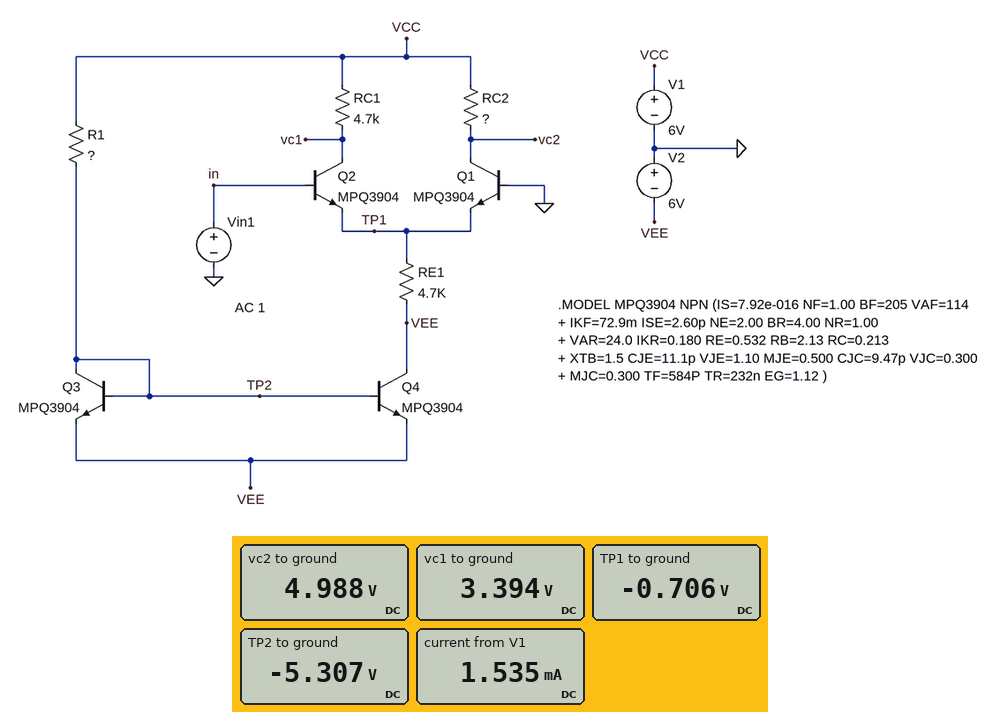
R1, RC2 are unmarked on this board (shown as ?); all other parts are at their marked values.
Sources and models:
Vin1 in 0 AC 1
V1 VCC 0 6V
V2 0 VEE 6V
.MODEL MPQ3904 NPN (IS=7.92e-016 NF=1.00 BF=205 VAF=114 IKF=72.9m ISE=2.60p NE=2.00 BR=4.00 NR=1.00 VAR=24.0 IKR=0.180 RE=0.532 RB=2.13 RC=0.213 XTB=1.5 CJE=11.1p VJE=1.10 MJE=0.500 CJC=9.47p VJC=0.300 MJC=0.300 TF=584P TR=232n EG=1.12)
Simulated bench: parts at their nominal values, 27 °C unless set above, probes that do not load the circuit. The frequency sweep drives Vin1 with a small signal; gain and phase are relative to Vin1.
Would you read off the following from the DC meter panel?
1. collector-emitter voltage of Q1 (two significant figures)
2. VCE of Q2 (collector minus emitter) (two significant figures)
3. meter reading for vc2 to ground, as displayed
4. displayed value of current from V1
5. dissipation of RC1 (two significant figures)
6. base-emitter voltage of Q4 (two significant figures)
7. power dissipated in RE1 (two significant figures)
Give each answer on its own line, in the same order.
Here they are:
5.7 V
4.1 V
4.988 V
1.535 mA
1.4 mW
690 mV
6.0 mW
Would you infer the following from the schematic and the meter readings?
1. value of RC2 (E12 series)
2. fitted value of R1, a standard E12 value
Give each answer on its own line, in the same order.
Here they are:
1.8 kΩ
27 kΩ
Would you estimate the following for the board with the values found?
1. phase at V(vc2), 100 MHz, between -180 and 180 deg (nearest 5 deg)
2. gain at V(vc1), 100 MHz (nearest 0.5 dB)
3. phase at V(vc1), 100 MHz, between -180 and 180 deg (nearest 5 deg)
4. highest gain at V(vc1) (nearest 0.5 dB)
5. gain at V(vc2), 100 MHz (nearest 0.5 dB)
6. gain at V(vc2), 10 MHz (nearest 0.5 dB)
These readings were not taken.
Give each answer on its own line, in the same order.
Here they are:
-80 deg
11.5 dB
75 deg
34.0 dB
12.0 dB
24.5 dB
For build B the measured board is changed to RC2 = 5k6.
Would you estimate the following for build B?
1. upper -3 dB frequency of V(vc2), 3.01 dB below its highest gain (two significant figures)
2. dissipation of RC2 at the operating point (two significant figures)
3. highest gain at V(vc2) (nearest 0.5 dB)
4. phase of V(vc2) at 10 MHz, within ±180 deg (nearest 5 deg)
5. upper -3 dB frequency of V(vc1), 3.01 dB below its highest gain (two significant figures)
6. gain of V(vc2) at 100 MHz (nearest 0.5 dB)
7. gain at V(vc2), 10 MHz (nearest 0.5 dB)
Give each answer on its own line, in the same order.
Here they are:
6.0 MHz
1.7 mW
35.0 dB
-60 deg
7.4 MHz
10.5 dB
29.5 dB
